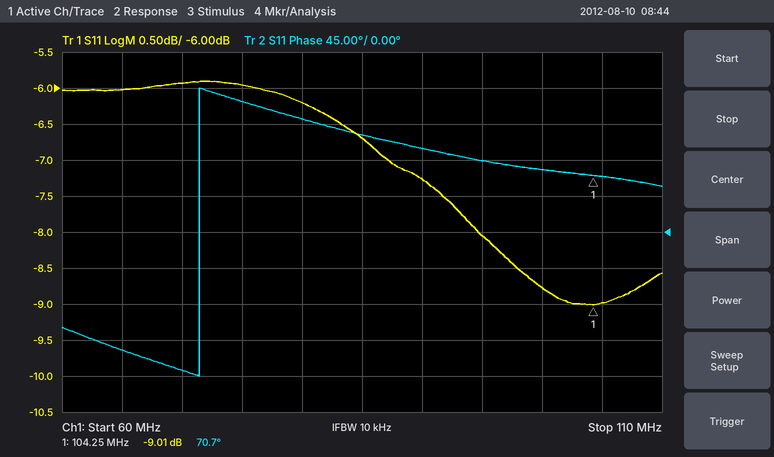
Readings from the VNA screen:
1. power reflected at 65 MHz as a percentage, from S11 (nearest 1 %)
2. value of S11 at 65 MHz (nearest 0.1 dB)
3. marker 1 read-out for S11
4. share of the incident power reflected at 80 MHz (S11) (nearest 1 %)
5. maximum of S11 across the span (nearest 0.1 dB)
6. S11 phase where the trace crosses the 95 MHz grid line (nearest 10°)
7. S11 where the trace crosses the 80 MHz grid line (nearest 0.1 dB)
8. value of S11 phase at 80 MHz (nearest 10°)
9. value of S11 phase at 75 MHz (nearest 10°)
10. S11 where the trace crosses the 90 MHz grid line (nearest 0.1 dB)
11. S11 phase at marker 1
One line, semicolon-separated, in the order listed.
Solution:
25 %; -6.0 dB; -9.01 dB; 24 %; -5.9 dB; 90°; -6.2 dB; 140°; 160°; -7.3 dB; 70.7°
